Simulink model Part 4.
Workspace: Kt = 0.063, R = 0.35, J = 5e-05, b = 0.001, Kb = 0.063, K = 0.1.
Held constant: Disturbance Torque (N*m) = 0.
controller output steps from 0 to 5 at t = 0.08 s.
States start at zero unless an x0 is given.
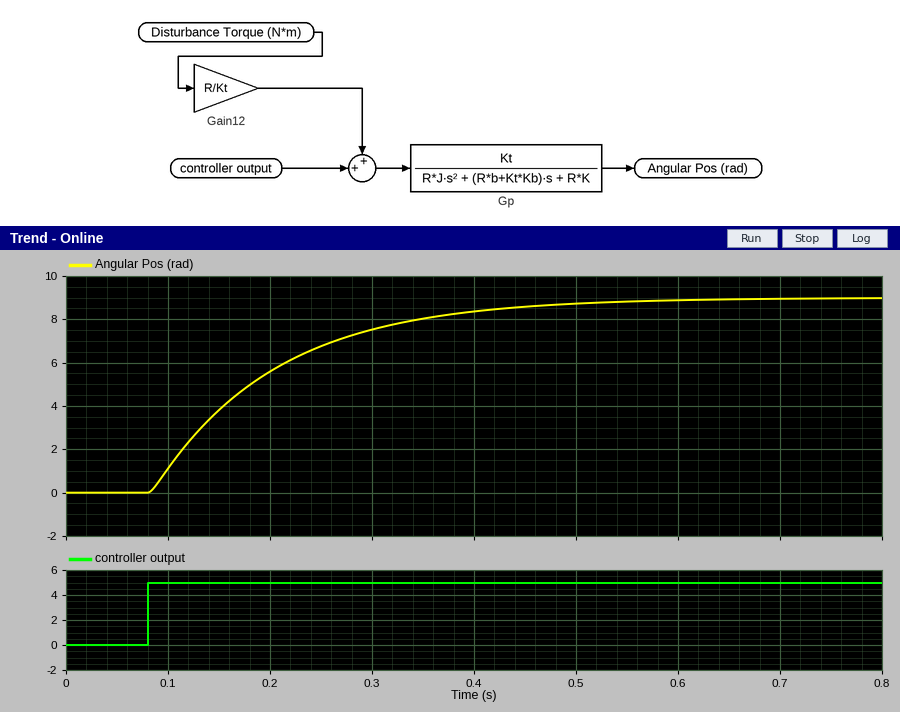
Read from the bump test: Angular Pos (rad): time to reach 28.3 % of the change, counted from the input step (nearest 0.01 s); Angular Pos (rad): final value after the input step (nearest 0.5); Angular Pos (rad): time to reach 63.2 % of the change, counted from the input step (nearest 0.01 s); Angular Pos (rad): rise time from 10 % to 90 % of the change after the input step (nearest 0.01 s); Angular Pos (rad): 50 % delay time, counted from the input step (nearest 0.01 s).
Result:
0.04 s
9.0
0.12 s
0.26 s
0.09 s
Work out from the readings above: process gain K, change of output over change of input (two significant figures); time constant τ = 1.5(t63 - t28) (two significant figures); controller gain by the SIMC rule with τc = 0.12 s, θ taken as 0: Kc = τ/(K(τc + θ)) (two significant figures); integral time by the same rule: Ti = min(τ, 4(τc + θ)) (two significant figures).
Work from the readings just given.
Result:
1.8
0.12 s
0.56
0.12 s
